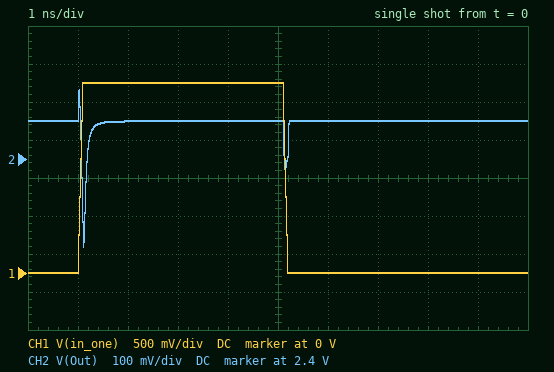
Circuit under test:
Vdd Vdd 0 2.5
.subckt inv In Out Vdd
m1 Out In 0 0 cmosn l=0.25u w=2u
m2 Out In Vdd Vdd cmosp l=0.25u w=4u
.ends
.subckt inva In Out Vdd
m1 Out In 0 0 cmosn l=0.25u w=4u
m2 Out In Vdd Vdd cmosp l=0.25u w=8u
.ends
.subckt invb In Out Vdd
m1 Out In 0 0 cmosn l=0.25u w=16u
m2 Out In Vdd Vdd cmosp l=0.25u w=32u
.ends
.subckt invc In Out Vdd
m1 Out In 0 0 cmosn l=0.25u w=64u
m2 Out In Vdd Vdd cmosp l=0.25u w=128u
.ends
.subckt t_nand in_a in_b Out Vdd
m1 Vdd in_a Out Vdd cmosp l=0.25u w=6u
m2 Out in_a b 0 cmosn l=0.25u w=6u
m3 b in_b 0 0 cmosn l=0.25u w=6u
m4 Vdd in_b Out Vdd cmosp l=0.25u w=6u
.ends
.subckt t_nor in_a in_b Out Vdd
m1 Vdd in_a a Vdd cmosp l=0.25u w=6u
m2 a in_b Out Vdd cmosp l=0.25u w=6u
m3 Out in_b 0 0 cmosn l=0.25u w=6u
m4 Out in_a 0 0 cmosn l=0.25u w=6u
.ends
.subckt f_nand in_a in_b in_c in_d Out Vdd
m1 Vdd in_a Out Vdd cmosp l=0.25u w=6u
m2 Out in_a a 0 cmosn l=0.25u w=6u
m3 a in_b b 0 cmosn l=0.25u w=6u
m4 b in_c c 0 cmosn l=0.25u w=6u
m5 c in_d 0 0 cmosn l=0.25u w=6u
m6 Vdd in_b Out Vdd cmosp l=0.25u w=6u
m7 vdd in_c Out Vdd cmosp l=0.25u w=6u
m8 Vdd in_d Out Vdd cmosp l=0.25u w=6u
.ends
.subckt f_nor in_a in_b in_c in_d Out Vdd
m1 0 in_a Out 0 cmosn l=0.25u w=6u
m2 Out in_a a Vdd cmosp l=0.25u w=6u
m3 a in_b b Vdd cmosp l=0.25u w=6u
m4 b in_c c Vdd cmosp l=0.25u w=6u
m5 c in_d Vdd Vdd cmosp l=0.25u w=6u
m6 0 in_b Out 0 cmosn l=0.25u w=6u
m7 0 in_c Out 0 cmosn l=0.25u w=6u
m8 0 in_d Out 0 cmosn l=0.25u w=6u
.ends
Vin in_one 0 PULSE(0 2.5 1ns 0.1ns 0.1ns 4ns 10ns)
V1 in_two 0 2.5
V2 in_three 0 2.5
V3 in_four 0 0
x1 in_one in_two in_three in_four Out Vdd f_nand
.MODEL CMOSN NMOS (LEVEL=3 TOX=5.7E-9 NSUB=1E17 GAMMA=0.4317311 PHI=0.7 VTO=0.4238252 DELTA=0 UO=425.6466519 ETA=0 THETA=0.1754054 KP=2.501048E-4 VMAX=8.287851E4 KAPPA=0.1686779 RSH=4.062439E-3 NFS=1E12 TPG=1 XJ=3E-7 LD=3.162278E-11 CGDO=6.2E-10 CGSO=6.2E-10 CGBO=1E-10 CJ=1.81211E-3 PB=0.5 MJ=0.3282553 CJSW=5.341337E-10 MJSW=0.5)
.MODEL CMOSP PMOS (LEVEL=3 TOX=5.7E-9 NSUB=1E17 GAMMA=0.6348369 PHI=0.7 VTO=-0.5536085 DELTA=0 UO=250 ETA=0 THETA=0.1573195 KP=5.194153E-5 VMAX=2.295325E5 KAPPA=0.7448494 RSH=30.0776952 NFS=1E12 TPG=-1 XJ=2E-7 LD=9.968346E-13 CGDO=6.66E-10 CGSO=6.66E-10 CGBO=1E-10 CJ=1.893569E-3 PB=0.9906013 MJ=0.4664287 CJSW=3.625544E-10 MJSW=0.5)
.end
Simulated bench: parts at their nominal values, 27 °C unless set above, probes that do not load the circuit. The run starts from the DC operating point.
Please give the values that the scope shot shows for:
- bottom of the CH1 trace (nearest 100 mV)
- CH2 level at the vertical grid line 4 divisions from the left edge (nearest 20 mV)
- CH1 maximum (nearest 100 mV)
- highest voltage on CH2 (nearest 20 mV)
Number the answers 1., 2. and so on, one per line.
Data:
1. 0 V
2. 2.50 V
3. 2.5 V
4. 2.58 V
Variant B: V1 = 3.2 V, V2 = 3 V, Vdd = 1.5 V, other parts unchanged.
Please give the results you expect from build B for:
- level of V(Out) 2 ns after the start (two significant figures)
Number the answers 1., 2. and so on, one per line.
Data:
1. 1.5 V
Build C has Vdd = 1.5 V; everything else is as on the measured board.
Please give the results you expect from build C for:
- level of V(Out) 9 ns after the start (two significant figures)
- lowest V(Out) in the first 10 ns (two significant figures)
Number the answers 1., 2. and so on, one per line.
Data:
1. 1.5 V
2. 1.3 V
